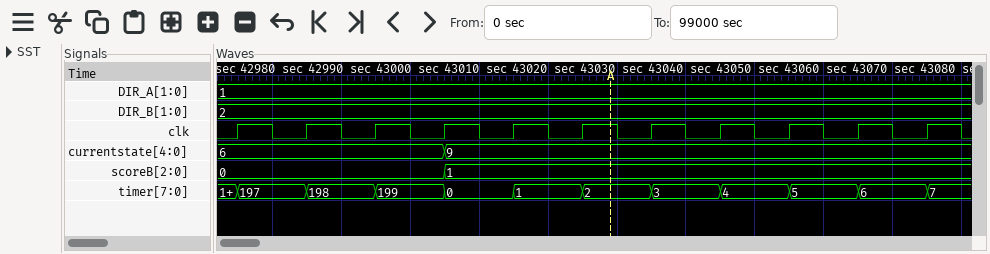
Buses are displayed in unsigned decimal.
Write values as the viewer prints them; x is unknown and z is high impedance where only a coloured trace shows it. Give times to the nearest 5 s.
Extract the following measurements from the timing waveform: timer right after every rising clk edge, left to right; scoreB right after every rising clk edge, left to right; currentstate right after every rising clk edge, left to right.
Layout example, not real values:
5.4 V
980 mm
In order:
197, 198, 199, 0, 1, 2, 3, 4, 5, 6, 7
0, 0, 0, 1, 1, 1, 1, 1, 1, 1, 1
6, 6, 6, 9, 9, 9, 9, 9, 9, 9, 9
